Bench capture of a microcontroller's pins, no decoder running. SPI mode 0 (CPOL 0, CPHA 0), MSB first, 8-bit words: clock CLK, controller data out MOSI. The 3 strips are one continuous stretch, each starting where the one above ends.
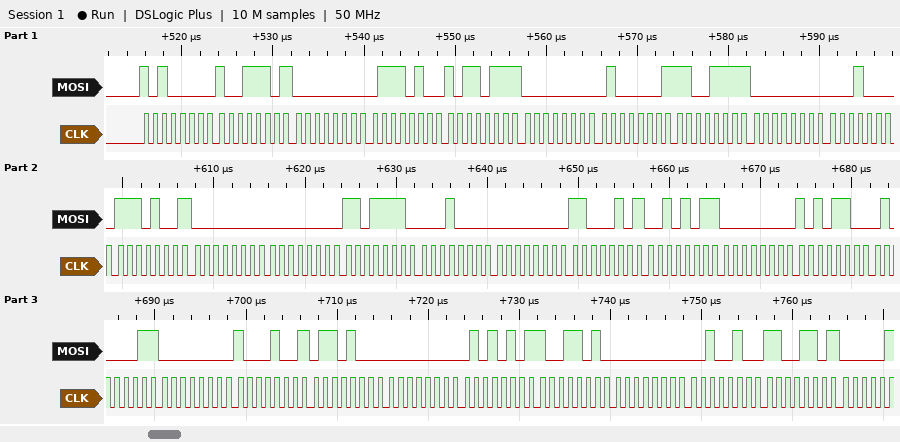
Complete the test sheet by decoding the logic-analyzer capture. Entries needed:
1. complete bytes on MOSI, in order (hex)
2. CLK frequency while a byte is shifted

A0 9D 00 74 B7 00 41 CF 00 10 E9 00 00 DE 10 00 C5 2B 00 AC 43 00 89 68 00 55 9A 00 24 CD
1 MHz
